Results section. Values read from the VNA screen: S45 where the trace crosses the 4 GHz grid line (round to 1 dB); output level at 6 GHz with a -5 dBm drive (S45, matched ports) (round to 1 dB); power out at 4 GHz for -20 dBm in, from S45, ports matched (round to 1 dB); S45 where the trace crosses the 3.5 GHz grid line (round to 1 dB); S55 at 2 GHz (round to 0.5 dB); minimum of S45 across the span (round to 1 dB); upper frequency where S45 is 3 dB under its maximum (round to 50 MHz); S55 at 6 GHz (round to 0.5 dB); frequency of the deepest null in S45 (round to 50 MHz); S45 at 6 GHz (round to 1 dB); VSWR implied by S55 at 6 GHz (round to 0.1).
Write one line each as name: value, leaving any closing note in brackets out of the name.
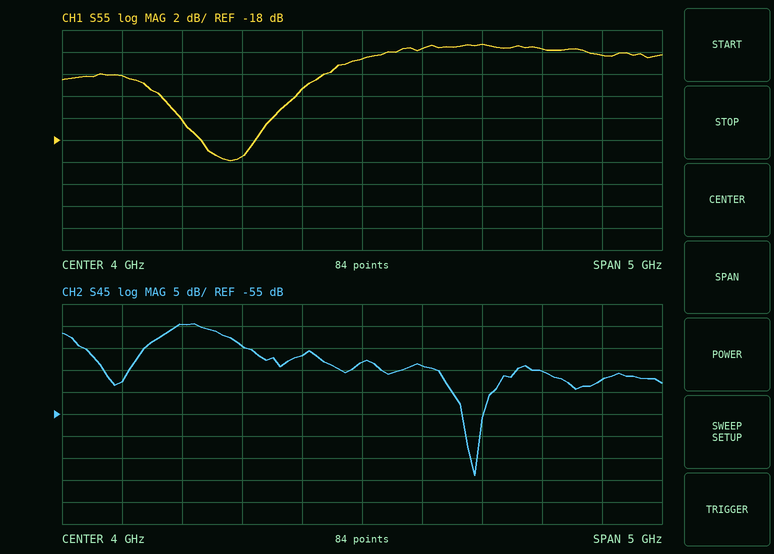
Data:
S45 where the trace crosses the 4 GHz grid line: -43 dB
output level at 6 GHz with a -5 dBm drive (S45, matched ports): -52 dBm
power out at 4 GHz for -20 dBm in, from S45, ports matched: -63 dBm
S45 where the trace crosses the 3.5 GHz grid line: -42 dB
S55 at 2 GHz: -12.0 dB
minimum of S45 across the span: -69 dB
upper frequency where S45 is 3 dB under its maximum: 2.90 GHz
S55 at 6 GHz: -10.5 dB
frequency of the deepest null in S45: 4.95 GHz
S45 at 6 GHz: -47 dB
VSWR implied by S55 at 6 GHz: 1.9
